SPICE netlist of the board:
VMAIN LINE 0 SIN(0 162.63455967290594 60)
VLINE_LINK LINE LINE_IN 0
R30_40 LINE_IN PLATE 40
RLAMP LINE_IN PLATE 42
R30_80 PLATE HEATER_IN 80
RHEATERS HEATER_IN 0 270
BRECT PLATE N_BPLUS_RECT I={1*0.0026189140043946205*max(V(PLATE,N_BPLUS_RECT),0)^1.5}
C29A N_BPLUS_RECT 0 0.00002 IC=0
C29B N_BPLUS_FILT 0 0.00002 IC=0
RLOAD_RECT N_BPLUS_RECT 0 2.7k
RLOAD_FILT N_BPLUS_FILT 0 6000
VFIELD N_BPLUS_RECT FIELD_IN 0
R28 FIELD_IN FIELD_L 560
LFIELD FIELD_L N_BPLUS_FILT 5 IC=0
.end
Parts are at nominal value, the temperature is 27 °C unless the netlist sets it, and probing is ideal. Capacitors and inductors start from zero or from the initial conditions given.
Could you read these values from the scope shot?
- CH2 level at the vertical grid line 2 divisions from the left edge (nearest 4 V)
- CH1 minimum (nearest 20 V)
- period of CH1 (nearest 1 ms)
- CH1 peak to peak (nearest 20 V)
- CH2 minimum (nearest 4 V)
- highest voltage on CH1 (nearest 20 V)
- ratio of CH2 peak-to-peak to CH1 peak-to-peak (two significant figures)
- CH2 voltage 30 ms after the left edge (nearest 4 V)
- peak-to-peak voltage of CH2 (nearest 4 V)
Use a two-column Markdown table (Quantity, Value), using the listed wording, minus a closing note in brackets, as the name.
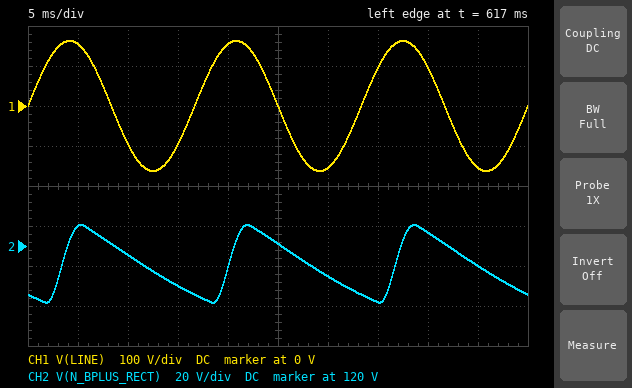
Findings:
| Quantity | Value |
|---|---|
| CH2 level at the vertical grid line 2 divisions from the left edge | 116 V |
| CH1 minimum | -160 V |
| period of CH1 | 17 ms |
| CH1 peak to peak | 320 V |
| CH2 minimum | 92 V |
| highest voltage on CH1 | 160 V |
| ratio of CH2 peak-to-peak to CH1 peak-to-peak | 0.12 |
| CH2 voltage 30 ms after the left edge | 104 V |
| peak-to-peak voltage of CH2 | 40 V |
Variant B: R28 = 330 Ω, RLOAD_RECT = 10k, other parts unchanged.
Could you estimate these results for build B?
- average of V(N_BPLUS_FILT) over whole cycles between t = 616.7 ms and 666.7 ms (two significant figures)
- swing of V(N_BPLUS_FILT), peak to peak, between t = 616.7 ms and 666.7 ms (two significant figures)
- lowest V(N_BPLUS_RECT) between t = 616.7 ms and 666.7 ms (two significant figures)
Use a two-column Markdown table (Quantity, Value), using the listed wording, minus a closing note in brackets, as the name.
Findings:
| Quantity | Value |
|---|---|
| average of V(N_BPLUS_FILT) over whole cycles between t = 616.7 ms and 666.7 ms | 120 V |
| swing of V(N_BPLUS_FILT), peak to peak, between t = 616.7 ms and 666.7 ms | 1.3 V |
| lowest V(N_BPLUS_RECT) between t = 616.7 ms and 666.7 ms | 110 V |
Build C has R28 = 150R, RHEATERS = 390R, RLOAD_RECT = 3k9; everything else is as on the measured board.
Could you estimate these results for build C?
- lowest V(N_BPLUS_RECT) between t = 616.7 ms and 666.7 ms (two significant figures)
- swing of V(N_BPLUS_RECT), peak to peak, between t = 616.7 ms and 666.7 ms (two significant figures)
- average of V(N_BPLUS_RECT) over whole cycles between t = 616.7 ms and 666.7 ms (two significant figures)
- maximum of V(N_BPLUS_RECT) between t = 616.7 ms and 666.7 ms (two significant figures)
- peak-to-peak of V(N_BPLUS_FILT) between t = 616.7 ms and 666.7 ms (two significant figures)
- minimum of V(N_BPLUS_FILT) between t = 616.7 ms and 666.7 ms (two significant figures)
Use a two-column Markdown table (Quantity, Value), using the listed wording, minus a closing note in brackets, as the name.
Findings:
| Quantity | Value |
|---|---|
| lowest V(N_BPLUS_RECT) between t = 616.7 ms and 666.7 ms | 100 V |
| swing of V(N_BPLUS_RECT), peak to peak, between t = 616.7 ms and 666.7 ms | 34 V |
| average of V(N_BPLUS_RECT) over whole cycles between t = 616.7 ms and 666.7 ms | 120 V |
| maximum of V(N_BPLUS_RECT) between t = 616.7 ms and 666.7 ms | 130 V |
| peak-to-peak of V(N_BPLUS_FILT) between t = 616.7 ms and 666.7 ms | 2.0 V |
| minimum of V(N_BPLUS_FILT) between t = 616.7 ms and 666.7 ms | 110 V |
